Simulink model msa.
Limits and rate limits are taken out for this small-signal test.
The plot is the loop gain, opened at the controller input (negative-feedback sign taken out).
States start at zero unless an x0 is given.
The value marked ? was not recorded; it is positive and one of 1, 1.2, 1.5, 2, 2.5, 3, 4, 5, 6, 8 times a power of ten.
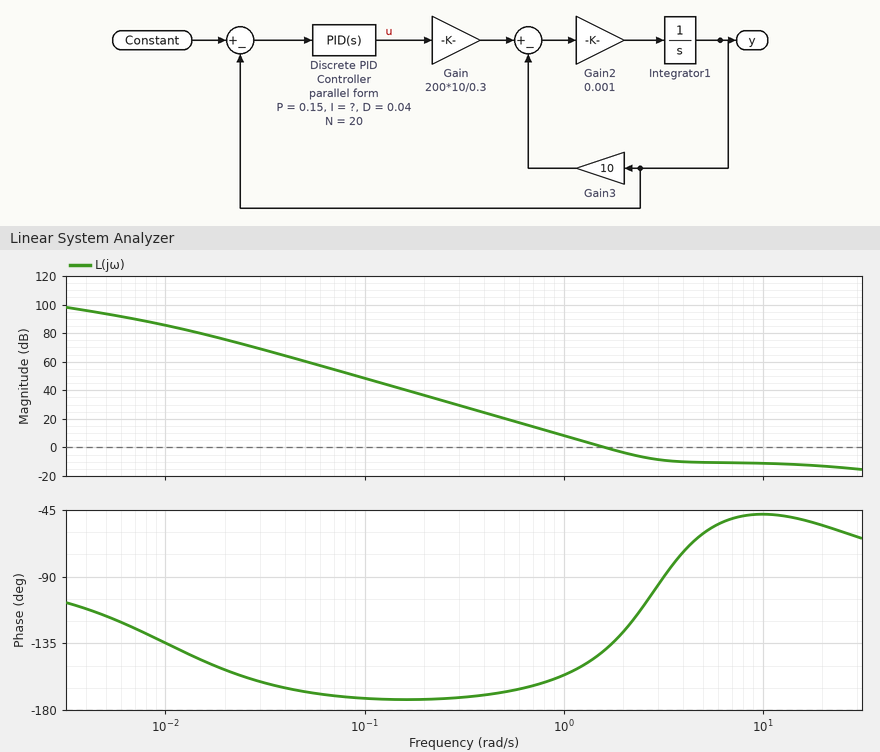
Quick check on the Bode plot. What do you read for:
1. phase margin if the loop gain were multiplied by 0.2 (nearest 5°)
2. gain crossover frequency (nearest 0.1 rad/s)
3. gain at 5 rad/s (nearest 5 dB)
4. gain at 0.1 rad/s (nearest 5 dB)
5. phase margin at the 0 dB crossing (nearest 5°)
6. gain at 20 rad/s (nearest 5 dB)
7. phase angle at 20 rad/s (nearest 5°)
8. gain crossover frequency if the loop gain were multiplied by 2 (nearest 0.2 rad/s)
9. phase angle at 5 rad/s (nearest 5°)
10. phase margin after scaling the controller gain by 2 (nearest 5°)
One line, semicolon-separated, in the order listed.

15°; 1.6 rad/s; -10 dB; 50 dB; 40°; -15 dB; -55°; 2.4 rad/s; -60°; 65°
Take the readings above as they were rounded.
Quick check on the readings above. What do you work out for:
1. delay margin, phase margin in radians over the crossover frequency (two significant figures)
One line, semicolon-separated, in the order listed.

0.44 s
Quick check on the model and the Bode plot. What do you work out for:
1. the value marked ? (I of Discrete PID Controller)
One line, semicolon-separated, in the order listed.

0.4
